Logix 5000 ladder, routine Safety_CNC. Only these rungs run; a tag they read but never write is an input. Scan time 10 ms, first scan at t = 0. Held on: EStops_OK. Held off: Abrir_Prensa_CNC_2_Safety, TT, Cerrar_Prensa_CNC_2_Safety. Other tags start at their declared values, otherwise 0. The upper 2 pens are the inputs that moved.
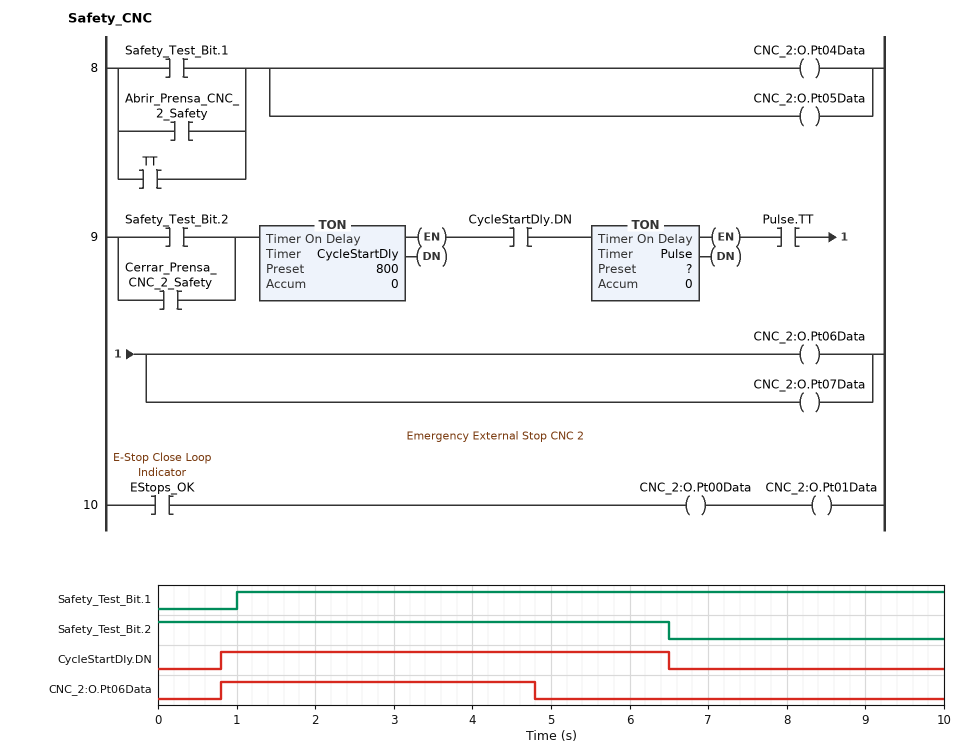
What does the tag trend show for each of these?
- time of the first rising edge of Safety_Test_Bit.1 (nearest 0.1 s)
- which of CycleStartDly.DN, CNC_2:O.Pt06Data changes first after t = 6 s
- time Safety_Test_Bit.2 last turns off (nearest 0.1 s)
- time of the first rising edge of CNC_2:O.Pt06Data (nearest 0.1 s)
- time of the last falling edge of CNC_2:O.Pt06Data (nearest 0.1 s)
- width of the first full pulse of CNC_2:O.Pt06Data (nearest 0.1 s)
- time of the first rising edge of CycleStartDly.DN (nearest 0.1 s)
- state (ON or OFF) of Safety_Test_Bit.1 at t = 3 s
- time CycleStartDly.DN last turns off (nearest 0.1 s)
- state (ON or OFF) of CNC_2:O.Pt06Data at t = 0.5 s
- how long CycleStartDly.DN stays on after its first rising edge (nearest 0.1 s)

1.0 s
CycleStartDly.DN
6.5 s
0.8 s
4.8 s
4.0 s
0.8 s
ON
6.5 s
OFF
5.7 s
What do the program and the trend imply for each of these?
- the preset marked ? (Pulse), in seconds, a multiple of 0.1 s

4.0 s
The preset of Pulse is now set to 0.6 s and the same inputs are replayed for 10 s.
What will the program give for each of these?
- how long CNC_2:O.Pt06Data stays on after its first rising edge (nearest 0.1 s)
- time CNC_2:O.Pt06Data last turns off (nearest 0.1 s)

0.6 s
1.4 s
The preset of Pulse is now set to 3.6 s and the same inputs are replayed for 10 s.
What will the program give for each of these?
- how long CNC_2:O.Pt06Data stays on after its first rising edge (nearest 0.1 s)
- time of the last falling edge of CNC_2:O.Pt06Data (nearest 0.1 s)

3.6 s
4.4 s
